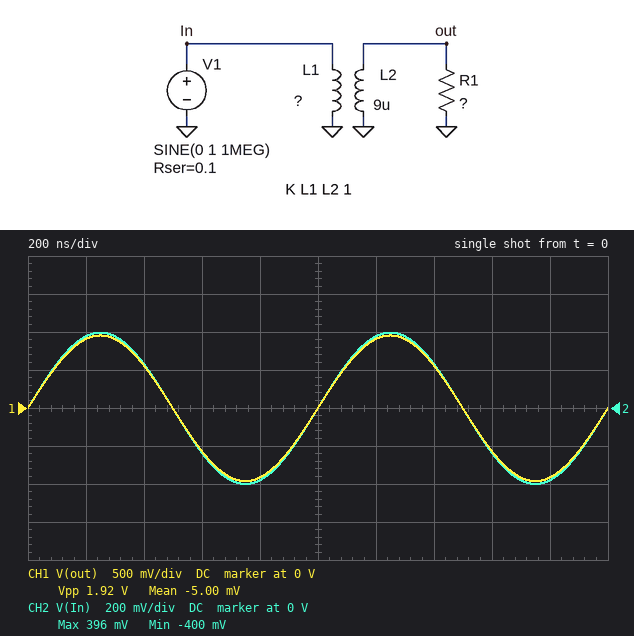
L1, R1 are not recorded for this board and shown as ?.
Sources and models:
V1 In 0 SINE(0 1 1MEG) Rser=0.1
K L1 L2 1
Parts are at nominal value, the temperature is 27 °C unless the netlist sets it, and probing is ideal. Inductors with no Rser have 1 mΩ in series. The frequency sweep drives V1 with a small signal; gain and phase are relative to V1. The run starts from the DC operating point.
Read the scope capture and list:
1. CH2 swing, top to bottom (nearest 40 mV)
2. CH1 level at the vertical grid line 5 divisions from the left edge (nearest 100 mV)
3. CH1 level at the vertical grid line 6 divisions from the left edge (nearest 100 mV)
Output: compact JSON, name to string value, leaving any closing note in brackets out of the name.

{"CH2 swing, top to bottom": "800 mV", "CH1 level at the vertical grid line 5 divisions from the left edge": "0 V", "CH1 level at the vertical grid line 6 divisions from the left edge": "900 mV"}
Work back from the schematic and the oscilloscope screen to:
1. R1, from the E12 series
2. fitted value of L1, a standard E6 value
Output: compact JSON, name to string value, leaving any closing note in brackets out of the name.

{"R1, from the E12 series": "0.39 Ω", "fitted value of L1, a standard E6 value": "1.5 µH"}
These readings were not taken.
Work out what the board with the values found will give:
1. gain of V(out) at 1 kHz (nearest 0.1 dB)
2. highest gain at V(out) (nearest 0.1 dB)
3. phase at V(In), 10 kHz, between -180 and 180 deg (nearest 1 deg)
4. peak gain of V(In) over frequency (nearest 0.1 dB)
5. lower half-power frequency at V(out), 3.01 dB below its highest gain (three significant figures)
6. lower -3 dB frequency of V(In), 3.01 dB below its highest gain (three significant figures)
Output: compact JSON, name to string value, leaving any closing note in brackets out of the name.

{"gain of V(out) at 1 kHz": "-13.1 dB", "highest gain at V(out)": "-0.4 dB", "phase at V(In), 10 kHz, between -180 and 180 deg": "22 deg", "peak gain of V(In) over frequency": "-8.0 dB", "lower half-power frequency at V(out), 3.01 dB below its highest gain": "4.20 kHz", "lower -3 dB frequency of V(In), 3.01 dB below its highest gain": "4.20 kHz"}
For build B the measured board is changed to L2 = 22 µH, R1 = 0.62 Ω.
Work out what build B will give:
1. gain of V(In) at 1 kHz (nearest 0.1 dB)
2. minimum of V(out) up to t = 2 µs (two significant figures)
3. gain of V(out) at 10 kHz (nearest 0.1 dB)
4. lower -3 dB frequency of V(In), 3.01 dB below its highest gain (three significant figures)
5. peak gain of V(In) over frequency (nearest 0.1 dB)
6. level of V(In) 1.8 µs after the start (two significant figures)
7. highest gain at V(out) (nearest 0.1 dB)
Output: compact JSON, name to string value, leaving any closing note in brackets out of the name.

{"gain of V(In) at 1 kHz": "-20.8 dB", "minimum of V(out) up to t = 2 µs": "-1.1 V", "gain of V(out) at 10 kHz": "0.6 dB", "lower -3 dB frequency of V(In), 3.01 dB below its highest gain": "3.16 kHz", "peak gain of V(In) over frequency": "-10.4 dB", "level of V(In) 1.8 µs after the start": "-290 mV", "highest gain at V(out)": "1.1 dB"}
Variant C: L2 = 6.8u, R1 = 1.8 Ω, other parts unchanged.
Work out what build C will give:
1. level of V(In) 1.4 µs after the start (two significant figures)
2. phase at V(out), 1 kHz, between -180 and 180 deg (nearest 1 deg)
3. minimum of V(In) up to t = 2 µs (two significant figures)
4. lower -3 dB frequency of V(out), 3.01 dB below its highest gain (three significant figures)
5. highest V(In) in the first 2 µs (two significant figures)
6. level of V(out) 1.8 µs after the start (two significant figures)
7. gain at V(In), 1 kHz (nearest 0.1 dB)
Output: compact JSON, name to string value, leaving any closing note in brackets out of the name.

{"level of V(In) 1.4 µs after the start": "460 mV", "phase at V(out), 1 kHz, between -180 and 180 deg": "83 deg", "minimum of V(In) up to t = 2 µs": "-810 mV", "lower -3 dB frequency of V(out), 3.01 dB below its highest gain": "8.54 kHz", "highest V(In) in the first 2 µs": "790 mV", "level of V(out) 1.8 µs after the start": "-1.6 V", "gain at V(In), 1 kHz": "-20.6 dB"}
